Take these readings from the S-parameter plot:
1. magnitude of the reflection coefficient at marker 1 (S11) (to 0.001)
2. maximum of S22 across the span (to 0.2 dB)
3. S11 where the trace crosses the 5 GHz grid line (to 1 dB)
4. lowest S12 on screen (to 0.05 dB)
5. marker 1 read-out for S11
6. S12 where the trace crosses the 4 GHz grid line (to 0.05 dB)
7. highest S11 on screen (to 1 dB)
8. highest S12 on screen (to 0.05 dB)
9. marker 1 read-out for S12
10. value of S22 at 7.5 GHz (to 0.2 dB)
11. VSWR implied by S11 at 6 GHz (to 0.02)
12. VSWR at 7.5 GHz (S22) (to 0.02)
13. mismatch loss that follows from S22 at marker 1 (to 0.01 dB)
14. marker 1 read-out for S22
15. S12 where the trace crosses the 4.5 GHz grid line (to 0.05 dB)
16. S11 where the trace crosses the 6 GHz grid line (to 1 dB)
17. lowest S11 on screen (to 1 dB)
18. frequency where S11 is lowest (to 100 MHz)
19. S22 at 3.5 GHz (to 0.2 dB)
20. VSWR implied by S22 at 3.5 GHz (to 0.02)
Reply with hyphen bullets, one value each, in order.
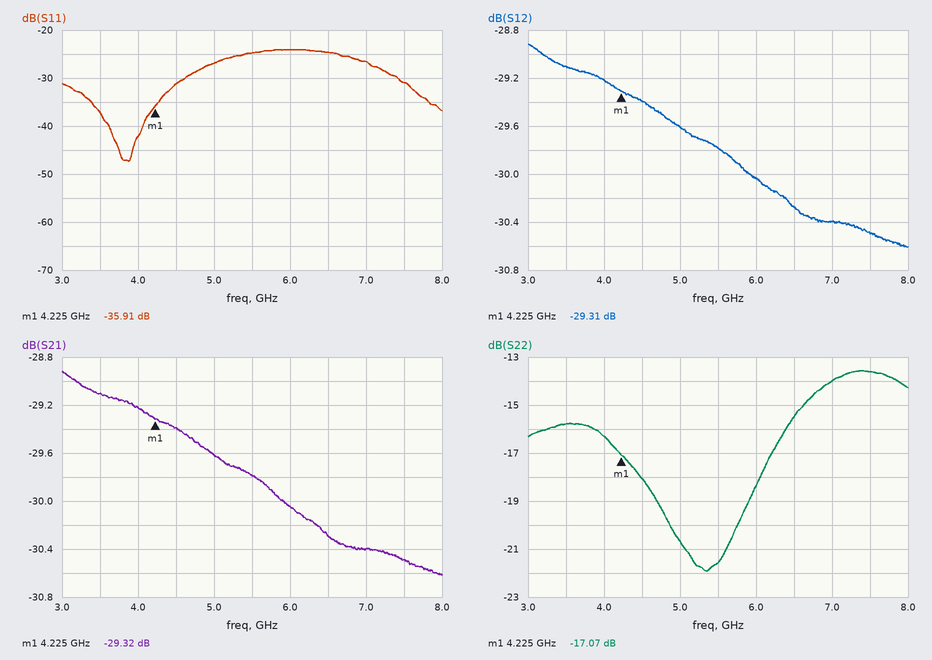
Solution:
- 0.016
- -13.6 dB
- -27 dB
- -30.60 dB
- -35.91 dB
- -29.20 dB
- -24 dB
- -28.90 dB
- -29.31 dB
- -13.6 dB
- 1.14
- 1.52
- 0.09 dB
- -17.07 dB
- -29.40 dB
- -24 dB
- -47 dB
- 3.9 GHz
- -15.8 dB
- 1.38
